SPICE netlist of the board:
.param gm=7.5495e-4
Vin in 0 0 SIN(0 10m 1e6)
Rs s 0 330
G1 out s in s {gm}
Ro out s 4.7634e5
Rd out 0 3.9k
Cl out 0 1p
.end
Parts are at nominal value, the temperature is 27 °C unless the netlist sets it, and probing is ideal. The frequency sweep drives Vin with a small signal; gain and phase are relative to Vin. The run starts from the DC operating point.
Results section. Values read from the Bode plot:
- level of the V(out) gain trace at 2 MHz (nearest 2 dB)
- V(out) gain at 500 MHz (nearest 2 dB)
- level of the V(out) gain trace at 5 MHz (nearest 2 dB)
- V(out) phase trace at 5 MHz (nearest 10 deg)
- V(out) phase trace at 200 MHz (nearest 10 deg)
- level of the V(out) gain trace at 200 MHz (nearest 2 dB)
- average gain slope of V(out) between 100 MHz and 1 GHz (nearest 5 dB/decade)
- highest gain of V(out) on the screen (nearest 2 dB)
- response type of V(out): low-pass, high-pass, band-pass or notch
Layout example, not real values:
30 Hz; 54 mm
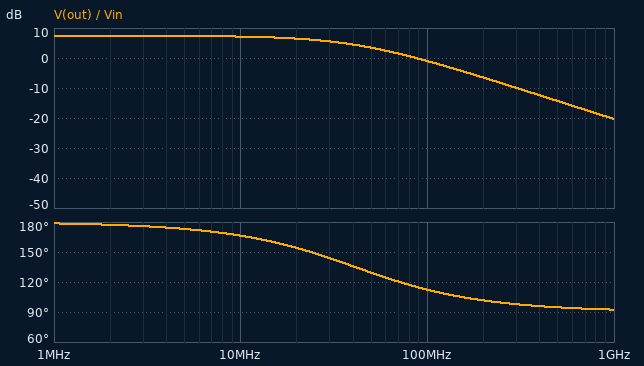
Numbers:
8 dB; -14 dB; 8 dB; 170 deg; 100 deg; -6 dB; -20 dB/decade; 8 dB; low-pass
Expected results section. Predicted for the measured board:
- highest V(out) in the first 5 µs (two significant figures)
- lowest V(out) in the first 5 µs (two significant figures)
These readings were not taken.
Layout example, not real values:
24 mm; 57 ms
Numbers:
23 mV; -23 mV
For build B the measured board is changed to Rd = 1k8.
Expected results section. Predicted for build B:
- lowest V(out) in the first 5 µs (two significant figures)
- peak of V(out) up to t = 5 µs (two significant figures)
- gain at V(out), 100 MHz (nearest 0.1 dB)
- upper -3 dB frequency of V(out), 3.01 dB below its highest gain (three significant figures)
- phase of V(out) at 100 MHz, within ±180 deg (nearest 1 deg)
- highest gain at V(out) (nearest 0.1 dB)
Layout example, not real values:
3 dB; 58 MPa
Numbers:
-11 mV; 11 mV; -2.9 dB; 88.7 MHz; 132 deg; 0.7 dB
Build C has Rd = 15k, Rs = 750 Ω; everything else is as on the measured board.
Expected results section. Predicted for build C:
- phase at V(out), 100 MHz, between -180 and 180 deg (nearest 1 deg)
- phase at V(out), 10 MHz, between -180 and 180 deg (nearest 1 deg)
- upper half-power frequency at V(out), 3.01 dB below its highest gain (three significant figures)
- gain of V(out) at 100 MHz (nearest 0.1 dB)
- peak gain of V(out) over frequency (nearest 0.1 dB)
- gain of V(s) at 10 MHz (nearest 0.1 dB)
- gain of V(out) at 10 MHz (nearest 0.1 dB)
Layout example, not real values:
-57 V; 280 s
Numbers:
96 deg; 137 deg; 10.8 MHz; -2.4 dB; 17.0 dB; -8.9 dB; 14.3 dB
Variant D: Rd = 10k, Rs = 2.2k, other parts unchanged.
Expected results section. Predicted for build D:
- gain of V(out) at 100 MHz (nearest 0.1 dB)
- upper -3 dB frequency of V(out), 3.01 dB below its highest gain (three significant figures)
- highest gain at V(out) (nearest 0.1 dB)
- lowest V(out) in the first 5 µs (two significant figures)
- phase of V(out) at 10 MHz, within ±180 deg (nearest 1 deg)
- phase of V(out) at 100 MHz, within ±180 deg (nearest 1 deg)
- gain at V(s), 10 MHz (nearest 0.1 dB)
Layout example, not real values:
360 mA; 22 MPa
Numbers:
-7.0 dB; 16.0 MHz; 9.0 dB; -28 mV; 148 deg; 99 deg; -4.2 dB
